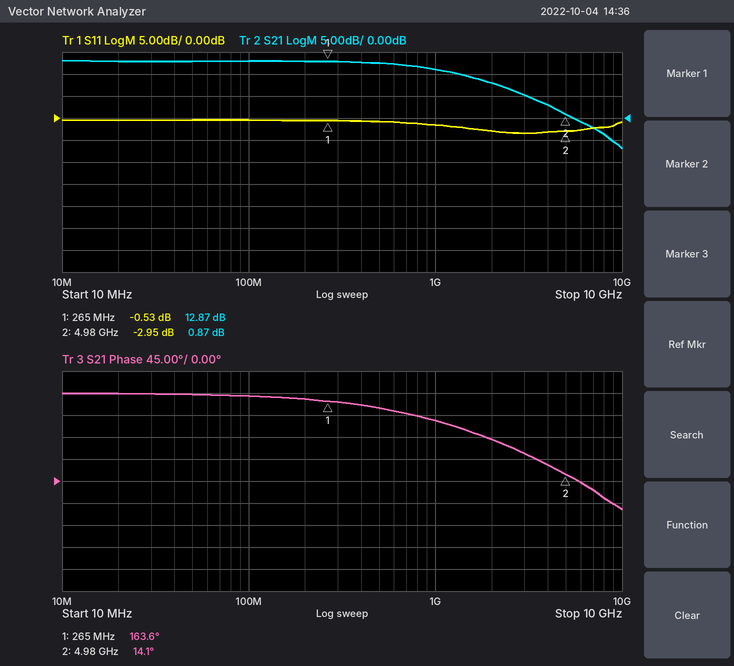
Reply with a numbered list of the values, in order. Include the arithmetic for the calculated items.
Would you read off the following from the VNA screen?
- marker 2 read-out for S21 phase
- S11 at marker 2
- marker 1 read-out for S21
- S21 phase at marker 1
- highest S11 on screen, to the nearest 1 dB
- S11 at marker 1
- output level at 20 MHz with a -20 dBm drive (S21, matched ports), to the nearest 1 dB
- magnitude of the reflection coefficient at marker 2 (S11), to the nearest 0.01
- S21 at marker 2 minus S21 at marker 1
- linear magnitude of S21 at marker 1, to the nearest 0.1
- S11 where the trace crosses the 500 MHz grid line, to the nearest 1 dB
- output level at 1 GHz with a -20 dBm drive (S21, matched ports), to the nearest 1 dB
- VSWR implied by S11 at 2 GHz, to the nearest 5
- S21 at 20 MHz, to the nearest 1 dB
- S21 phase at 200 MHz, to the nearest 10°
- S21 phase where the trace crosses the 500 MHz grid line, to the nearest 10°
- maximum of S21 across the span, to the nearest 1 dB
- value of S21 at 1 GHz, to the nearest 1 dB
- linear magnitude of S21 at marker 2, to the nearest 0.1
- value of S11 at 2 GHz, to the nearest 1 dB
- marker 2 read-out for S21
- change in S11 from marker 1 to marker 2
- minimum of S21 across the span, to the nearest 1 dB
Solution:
1. 14.1°
2. -2.95 dB
3. 12.87 dB
4. 163.6°
5. 0 dB
6. -0.53 dB
7. -20 dBm + (13 dB) = -7 dBm
8. 10^(-2.95/20) ≈ 0.71
9. 0.87 − (12.87) = -12.00 dB
10. 10^(12.87/20) ≈ 4.4
11. -1 dB
12. -20 dBm + (11 dB) = -9 dBm
13. |Γ| = 10^(-3/20) = 0.7079; VSWR = (1 + 0.7079)/(1 − 0.7079) ≈ 5.85, so 5 to the nearest 5
14. 13 dB
15. 170°
16. 150°
17. 13 dB
18. 11 dB
19. 10^(0.87/20) ≈ 1.1
20. -3 dB
21. 0.87 dB
22. -2.95 − (-0.53) = -2.42 dB
23. -7 dB
